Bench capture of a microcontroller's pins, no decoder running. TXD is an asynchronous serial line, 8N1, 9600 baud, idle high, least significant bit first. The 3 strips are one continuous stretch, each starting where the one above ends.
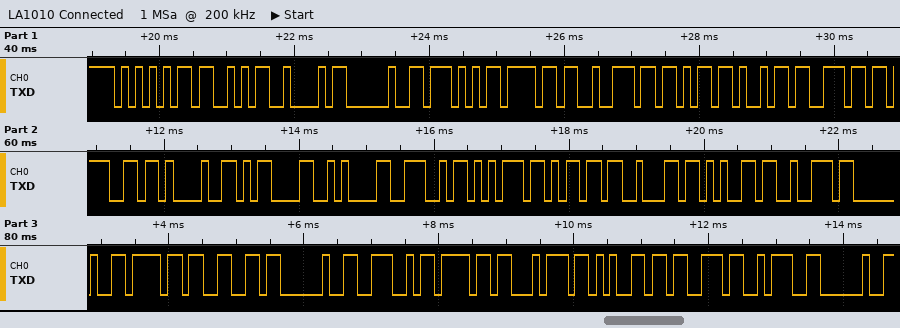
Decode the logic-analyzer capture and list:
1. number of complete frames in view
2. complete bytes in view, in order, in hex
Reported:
31
55 53 42 20 57 6F 72 6B 69 6E 67 21 0D 0A 4E 75 6D 62 65 72 20 6F 66 20 4E 6F 74 65 73 3A 20
